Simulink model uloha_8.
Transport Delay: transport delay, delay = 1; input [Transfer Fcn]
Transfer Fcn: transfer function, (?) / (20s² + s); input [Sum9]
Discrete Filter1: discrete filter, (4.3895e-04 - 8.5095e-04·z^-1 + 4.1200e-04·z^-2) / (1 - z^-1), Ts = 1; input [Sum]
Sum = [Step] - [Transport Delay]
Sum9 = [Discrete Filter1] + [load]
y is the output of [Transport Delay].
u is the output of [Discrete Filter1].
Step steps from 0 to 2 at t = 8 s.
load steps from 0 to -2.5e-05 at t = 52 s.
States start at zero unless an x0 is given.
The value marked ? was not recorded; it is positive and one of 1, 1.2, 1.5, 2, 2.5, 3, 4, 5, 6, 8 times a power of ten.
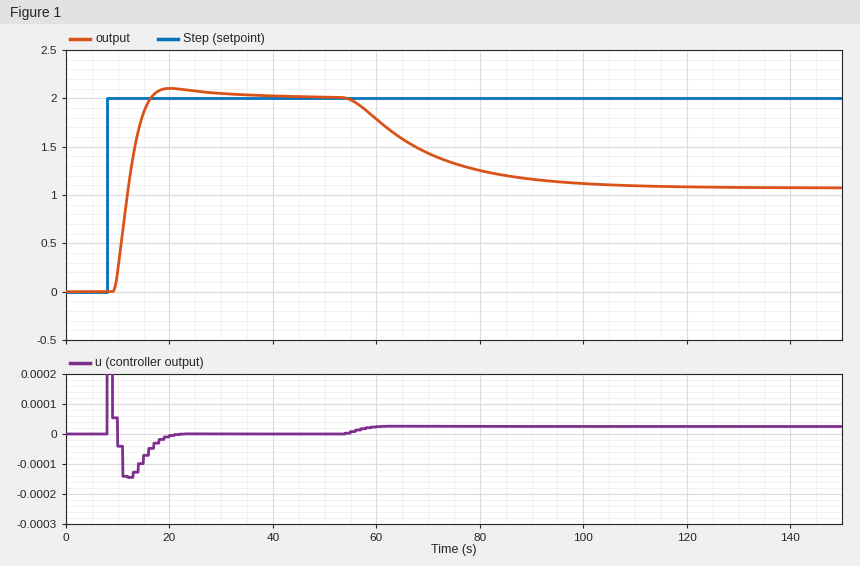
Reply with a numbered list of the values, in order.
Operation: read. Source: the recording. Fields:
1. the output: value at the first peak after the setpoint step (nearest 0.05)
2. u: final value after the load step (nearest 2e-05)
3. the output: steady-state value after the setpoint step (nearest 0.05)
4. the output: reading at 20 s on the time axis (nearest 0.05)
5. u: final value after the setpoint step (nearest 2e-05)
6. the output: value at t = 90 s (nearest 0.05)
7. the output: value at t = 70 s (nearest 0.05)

1. 2.10
2. 0.00002
3. 2.00
4. 2.10
5. 0.00000
6. 1.15
7. 1.45
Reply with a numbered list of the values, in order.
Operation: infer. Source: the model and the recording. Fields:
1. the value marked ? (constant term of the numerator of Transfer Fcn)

1. 10000
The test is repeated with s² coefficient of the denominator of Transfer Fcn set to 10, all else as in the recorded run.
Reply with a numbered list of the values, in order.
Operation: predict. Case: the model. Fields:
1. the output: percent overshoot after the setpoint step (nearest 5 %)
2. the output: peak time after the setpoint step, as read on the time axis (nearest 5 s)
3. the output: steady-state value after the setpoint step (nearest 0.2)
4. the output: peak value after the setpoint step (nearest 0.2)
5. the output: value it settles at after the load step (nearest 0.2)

1. 25 %
2. 15 s
3. 2.0
4. 2.4
5. 1.0
